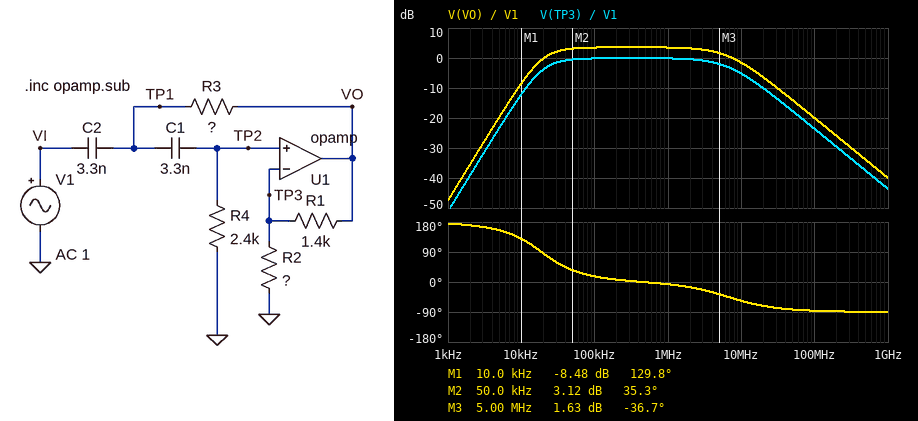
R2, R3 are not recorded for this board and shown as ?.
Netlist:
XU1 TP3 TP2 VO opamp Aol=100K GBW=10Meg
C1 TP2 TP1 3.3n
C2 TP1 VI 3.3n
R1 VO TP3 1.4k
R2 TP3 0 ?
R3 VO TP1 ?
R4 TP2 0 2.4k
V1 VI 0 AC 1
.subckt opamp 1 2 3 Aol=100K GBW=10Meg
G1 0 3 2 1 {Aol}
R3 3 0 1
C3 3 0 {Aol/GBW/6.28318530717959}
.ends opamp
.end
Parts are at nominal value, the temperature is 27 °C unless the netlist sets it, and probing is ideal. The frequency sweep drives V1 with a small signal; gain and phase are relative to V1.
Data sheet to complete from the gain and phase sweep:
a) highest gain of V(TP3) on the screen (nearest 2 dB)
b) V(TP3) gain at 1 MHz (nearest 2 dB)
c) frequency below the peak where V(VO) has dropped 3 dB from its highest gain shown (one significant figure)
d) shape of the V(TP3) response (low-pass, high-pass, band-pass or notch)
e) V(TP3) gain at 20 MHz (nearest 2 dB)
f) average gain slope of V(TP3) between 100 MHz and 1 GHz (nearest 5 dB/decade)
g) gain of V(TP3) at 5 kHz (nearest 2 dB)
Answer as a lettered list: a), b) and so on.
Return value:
a) 0 dB
b) 0 dB
c) 20 kHz
d) band-pass
e) -10 dB
f) -20 dB/decade
g) -24 dB
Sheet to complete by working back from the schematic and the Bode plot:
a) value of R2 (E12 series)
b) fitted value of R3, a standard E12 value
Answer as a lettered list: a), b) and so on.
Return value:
a) 2.7 kΩ
b) 2.7 kΩ
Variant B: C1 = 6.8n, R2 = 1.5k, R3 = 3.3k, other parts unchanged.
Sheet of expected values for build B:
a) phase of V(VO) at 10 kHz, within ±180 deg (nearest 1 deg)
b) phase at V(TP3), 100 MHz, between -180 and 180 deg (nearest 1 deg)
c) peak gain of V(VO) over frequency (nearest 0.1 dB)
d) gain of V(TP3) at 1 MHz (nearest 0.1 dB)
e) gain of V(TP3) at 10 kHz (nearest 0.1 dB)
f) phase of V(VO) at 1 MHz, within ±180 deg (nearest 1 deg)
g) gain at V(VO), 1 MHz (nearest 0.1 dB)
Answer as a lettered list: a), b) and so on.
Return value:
a) 104 deg
b) -87 deg
c) 5.7 dB
d) -0.2 dB
e) -4.5 dB
f) -10 deg
g) 5.5 dB
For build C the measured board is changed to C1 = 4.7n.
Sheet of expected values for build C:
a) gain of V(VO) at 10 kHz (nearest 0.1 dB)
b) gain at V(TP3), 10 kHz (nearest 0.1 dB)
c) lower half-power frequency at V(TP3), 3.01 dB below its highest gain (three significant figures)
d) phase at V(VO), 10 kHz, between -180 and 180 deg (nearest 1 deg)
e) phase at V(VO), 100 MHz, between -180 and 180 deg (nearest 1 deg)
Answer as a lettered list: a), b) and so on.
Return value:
a) -5.7 dB
b) -9.3 dB
c) 17.7 kHz
d) 121 deg
e) -86 deg
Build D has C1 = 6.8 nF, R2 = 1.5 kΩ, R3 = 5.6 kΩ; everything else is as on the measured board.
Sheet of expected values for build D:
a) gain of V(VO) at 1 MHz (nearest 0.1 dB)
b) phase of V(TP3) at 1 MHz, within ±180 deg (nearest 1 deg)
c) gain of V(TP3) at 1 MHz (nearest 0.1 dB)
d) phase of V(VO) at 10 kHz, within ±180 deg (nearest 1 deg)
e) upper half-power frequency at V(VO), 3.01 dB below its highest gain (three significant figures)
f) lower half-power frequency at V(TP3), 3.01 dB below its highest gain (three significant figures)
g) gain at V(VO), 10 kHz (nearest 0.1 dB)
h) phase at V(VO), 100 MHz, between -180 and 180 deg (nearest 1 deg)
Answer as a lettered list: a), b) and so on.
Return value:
a) 5.5 dB
b) -10 deg
c) -0.2 dB
d) 86 deg
e) 5.22 MHz
f) 18.0 kHz
g) -1.1 dB
h) -87 deg
